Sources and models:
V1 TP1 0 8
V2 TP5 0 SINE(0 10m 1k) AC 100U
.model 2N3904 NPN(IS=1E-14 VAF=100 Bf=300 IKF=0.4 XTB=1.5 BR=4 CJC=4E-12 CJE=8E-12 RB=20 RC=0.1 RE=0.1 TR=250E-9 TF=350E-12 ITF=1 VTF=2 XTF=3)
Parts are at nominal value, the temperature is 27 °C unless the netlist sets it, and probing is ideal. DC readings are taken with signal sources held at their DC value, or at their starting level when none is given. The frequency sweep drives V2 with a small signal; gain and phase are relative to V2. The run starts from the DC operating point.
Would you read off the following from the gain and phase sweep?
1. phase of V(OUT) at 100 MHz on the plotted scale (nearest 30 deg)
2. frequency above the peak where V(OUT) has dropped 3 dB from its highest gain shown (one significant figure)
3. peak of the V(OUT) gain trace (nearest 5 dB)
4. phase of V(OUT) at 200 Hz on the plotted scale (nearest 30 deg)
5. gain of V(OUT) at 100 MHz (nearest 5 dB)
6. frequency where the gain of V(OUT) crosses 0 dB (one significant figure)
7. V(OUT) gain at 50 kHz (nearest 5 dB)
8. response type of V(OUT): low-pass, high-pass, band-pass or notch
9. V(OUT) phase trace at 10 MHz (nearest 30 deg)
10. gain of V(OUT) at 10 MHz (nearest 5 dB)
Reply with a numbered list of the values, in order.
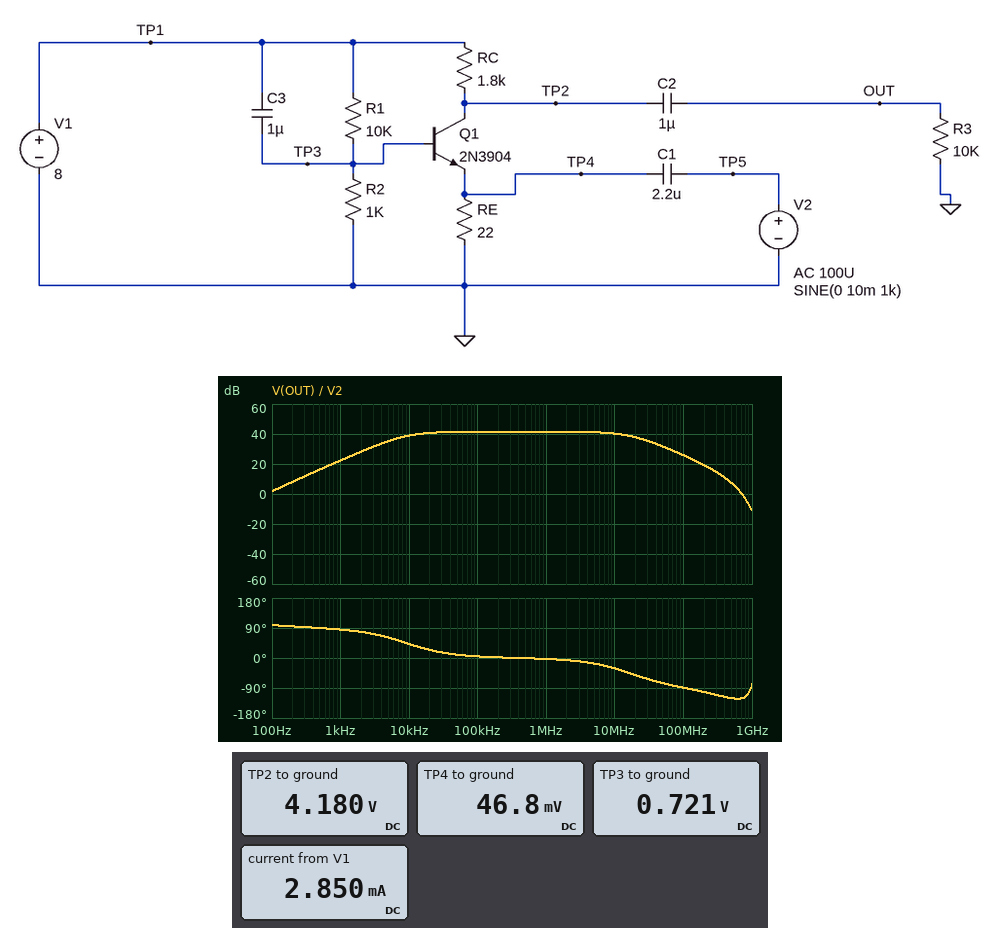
1. -90 deg
2. 20 MHz
3. 40 dB
4. 90 deg
5. 25 dB
6. 700 MHz
7. 40 dB
8. band-pass
9. -30 deg
10. 40 dB
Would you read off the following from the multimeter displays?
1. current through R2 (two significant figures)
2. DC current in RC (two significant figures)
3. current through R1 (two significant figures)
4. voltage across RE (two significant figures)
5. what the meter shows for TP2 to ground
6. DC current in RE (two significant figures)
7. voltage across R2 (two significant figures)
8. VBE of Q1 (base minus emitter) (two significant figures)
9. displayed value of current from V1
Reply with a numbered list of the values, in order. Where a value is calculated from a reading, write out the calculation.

1. (721 mV) / 1 kΩ = 720 µA
2. (8 V - 4.18 V) / 1.8 kΩ = 2.1 mA
3. (8 V - 721 mV) / 10 kΩ = 730 µA
4. 46.8 mV = 47 mV
5. 4.180 V
6. (46.8 mV) / 22 Ω = 2.1 mA
7. 721 mV = 720 mV
8. 721 mV - 46.8 mV = 670 mV
9. 2.850 mA
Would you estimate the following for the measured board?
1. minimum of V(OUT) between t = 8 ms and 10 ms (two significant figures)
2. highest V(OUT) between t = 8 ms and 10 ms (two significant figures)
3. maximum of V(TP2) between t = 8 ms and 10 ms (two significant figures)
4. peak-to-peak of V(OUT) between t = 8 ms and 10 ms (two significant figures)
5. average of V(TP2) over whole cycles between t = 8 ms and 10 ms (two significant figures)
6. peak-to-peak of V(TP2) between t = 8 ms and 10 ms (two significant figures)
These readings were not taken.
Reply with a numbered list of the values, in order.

1. -130 mV
2. 130 mV
3. 4.3 V
4. 260 mV
5. 4.2 V
6. 260 mV
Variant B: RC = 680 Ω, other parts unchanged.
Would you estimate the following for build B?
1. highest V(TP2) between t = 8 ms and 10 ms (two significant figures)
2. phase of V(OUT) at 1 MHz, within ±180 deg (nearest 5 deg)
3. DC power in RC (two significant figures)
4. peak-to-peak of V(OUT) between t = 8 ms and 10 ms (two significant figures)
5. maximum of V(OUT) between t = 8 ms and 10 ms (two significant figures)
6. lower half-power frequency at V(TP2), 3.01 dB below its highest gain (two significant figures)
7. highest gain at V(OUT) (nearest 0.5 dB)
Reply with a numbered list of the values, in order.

1. 6.6 V
2. 0 deg
3. 3.1 mW
4. 110 mV
5. 55 mV
6. 9.1 kHz
7. 34.0 dB
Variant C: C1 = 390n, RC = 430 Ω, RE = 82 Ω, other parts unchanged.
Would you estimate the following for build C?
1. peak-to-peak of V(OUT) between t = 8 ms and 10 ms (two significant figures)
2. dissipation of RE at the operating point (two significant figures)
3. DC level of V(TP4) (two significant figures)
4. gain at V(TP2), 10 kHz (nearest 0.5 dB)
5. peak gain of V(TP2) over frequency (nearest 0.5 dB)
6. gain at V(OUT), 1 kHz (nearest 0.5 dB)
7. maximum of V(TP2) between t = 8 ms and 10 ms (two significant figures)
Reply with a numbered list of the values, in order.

1. 15 mV
2. 67 µW
3. 74 mV
4. 16.5 dB
5. 23.0 dB
6. -2.5 dB
7. 7.6 V
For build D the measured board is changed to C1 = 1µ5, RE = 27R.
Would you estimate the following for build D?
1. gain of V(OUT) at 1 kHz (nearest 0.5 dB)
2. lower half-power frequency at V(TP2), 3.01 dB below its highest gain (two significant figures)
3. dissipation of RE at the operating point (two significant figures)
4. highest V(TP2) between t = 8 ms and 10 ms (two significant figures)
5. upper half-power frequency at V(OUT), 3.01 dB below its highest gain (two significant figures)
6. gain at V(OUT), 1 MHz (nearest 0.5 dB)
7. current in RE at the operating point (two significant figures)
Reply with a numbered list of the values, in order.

1. 19.5 dB
2. 11 kHz
3. 96 µW
4. 4.7 V
5. 19 MHz
6. 40.5 dB
7. 1.9 mA
